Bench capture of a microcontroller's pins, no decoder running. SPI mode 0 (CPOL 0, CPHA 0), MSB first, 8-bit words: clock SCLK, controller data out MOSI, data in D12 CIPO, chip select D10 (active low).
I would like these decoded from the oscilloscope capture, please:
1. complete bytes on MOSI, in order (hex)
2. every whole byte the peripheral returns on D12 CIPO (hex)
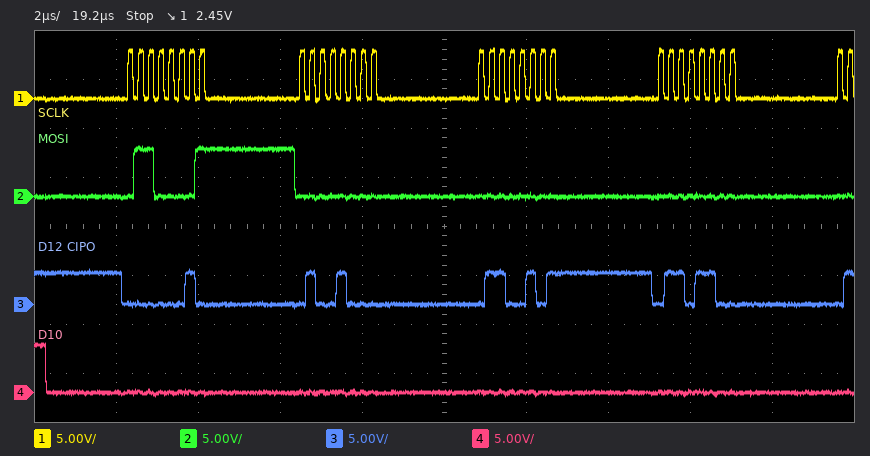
61 00 00 00
02 48 65 6C
